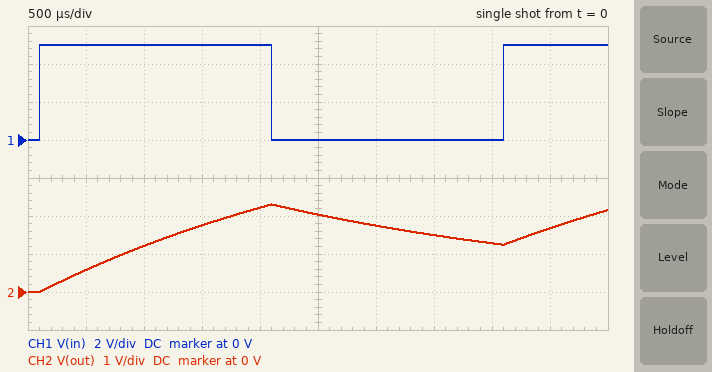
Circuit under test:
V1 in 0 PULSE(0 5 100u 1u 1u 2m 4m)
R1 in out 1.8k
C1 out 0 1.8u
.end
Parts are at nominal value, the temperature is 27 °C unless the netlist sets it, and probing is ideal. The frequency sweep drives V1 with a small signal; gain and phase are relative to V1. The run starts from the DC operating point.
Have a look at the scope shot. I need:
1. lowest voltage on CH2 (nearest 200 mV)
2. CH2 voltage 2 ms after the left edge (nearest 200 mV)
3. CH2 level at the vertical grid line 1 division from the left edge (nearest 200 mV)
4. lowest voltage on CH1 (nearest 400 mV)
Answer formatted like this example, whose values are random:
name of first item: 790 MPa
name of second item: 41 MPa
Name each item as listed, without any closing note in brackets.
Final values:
lowest voltage on CH2: 0 V
CH2 voltage 2 ms after the left edge: 2.2 V
CH2 level at the vertical grid line 1 division from the left edge: 600 mV
lowest voltage on CH1: 0 V
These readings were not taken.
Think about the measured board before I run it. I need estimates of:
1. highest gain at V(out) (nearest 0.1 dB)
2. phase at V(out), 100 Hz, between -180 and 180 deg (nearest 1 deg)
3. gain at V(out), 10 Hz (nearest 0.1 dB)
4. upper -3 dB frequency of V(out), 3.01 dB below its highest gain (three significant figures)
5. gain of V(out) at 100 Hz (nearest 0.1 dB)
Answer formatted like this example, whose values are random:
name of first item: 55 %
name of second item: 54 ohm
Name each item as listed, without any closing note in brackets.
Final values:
highest gain at V(out): 0 dB
phase at V(out), 100 Hz, between -180 and 180 deg: -64 deg
gain at V(out), 10 Hz: -0.2 dB
upper -3 dB frequency of V(out), 3.01 dB below its highest gain: 49.1 Hz
gain of V(out) at 100 Hz: -7.1 dB
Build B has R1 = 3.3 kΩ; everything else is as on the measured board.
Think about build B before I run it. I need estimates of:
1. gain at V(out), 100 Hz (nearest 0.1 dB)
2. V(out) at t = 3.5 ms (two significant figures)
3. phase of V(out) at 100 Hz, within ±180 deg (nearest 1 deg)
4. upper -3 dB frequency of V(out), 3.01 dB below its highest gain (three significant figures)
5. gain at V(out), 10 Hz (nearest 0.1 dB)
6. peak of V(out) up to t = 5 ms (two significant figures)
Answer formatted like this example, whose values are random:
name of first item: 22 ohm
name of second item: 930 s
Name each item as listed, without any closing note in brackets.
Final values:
gain at V(out), 100 Hz: -11.7 dB
V(out) at t = 3.5 ms: 1.1 V
phase of V(out) at 100 Hz, within ±180 deg: -75 deg
upper -3 dB frequency of V(out), 3.01 dB below its highest gain: 26.8 Hz
gain at V(out), 10 Hz: -0.6 dB
peak of V(out) up to t = 5 ms: 1.6 V
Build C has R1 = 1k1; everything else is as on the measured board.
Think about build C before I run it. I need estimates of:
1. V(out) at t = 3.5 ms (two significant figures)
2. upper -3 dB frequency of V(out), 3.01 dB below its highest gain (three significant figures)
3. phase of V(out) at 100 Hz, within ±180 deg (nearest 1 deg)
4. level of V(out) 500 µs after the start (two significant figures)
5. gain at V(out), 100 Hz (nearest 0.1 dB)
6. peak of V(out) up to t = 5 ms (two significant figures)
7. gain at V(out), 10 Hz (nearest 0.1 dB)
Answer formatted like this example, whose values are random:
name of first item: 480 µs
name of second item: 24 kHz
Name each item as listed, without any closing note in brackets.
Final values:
V(out) at t = 3.5 ms: 1.6 V
upper -3 dB frequency of V(out), 3.01 dB below its highest gain: 80.4 Hz
phase of V(out) at 100 Hz, within ±180 deg: -51 deg
level of V(out) 500 µs after the start: 910 mV
gain at V(out), 100 Hz: -4.1 dB
peak of V(out) up to t = 5 ms: 3.2 V
gain at V(out), 10 Hz: -0.1 dB
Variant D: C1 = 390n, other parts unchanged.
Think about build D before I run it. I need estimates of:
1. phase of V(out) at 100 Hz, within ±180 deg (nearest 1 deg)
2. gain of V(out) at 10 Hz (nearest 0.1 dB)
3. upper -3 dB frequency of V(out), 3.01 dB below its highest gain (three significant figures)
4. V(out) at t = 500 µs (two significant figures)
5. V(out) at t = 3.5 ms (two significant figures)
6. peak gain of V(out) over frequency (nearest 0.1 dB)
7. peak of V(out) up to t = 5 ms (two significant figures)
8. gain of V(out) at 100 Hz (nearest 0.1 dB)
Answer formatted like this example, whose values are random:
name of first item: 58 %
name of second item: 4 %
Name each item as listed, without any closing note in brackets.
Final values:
phase of V(out) at 100 Hz, within ±180 deg: -24 deg
gain of V(out) at 10 Hz: 0 dB
upper -3 dB frequency of V(out), 3.01 dB below its highest gain: 227 Hz
V(out) at t = 500 µs: 2.2 V
V(out) at t = 3.5 ms: 640 mV
peak gain of V(out) over frequency: 0 dB
peak of V(out) up to t = 5 ms: 4.7 V
gain of V(out) at 100 Hz: -0.8 dB
